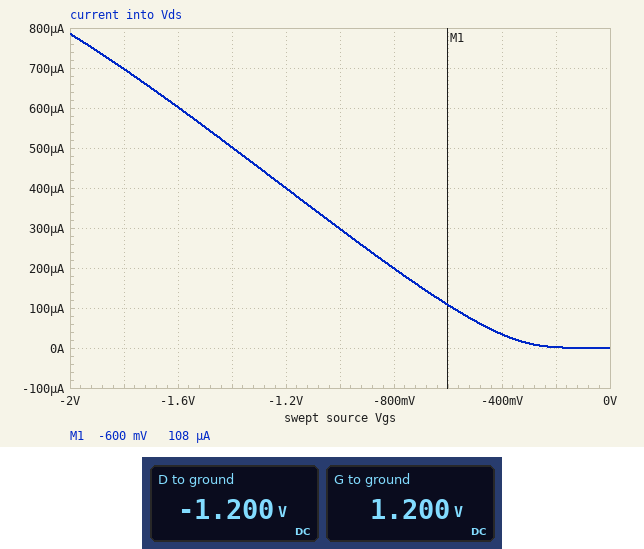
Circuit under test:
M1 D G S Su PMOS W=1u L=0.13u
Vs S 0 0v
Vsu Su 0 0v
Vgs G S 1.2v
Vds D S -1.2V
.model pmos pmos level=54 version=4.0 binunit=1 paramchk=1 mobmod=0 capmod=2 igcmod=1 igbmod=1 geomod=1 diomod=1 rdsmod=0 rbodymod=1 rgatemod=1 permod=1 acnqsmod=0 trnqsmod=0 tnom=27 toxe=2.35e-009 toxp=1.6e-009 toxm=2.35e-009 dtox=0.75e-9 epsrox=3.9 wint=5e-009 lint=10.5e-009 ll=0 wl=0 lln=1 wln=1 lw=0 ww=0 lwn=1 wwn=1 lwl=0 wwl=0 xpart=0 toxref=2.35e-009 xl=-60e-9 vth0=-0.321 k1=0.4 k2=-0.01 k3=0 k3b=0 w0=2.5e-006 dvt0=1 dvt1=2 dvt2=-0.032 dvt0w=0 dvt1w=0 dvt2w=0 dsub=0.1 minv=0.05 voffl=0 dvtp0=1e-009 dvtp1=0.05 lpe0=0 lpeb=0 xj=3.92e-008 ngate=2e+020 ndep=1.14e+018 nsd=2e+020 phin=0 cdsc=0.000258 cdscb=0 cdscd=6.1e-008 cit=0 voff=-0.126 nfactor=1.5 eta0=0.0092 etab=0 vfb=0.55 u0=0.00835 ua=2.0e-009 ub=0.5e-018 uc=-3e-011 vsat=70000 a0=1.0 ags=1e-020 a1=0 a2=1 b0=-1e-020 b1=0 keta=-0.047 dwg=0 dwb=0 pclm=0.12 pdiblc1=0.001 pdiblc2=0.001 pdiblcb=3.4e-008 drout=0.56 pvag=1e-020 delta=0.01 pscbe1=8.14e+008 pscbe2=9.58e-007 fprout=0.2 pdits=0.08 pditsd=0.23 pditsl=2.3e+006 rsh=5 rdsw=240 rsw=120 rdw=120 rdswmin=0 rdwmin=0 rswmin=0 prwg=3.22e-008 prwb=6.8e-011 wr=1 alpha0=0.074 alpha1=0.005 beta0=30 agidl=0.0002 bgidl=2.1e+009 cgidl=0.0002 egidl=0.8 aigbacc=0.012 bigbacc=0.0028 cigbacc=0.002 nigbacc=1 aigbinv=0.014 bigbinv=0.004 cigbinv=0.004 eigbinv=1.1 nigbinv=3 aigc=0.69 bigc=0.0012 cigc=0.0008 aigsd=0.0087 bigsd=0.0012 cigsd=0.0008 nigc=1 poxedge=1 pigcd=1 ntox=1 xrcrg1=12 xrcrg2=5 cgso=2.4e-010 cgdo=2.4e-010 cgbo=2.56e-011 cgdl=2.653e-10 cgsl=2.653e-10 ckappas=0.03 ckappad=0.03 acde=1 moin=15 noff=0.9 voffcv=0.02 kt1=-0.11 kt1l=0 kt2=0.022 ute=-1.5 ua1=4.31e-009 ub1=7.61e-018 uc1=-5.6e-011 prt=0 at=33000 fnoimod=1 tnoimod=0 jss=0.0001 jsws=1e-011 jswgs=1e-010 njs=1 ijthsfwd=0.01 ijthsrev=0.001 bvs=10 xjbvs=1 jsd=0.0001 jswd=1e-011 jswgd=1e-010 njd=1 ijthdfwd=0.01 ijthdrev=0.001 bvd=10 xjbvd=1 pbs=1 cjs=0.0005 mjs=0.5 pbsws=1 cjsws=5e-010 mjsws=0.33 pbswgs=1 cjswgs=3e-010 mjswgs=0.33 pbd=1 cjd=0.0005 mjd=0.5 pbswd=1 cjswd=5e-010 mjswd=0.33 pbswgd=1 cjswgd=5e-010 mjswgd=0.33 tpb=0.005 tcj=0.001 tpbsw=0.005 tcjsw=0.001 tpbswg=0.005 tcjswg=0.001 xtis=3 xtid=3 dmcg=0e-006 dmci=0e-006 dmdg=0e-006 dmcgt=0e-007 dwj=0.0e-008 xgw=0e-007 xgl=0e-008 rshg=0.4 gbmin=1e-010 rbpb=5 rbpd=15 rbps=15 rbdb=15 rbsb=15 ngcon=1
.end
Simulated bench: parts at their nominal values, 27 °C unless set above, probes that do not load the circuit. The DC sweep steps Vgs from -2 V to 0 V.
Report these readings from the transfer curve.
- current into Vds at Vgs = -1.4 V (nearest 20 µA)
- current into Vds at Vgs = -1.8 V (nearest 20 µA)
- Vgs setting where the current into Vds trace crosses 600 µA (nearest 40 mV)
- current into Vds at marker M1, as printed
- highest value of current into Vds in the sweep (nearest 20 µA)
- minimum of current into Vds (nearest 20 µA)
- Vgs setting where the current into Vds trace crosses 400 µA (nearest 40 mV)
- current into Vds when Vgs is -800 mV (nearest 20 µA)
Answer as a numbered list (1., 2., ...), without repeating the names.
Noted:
1. 500 µA
2. 700 µA
3. -1.60 V
4. 108 µA
5. 780 µA
6. 0 A
7. -1.20 V
8. 200 µA
